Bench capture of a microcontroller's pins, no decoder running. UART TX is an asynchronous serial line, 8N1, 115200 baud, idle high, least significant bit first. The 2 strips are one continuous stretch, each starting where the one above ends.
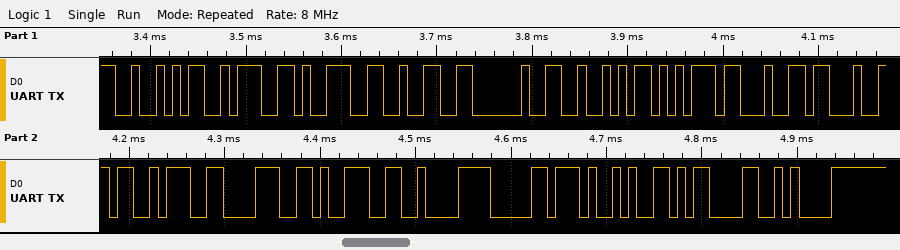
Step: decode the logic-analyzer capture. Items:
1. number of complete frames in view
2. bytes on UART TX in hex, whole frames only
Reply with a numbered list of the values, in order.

1. 17
2. 0x52 0x3A 0x39 0x32 0x20 0x52 0x75 0x64 0x64 0x3A 0x38 0x39 0xC2 0xB0 0x29 0x0D 0x0A
